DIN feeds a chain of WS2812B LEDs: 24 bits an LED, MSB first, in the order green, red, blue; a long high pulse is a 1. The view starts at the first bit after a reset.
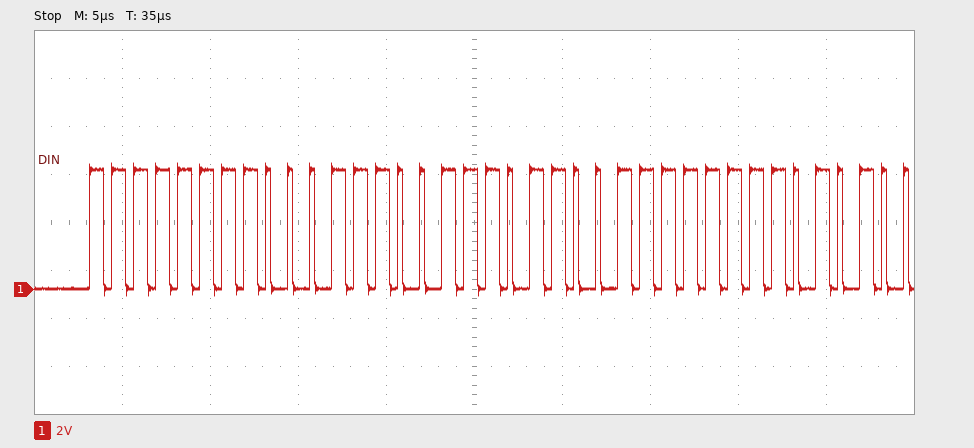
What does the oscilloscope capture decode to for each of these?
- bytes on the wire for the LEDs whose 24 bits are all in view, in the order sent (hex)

FF 1C EC
